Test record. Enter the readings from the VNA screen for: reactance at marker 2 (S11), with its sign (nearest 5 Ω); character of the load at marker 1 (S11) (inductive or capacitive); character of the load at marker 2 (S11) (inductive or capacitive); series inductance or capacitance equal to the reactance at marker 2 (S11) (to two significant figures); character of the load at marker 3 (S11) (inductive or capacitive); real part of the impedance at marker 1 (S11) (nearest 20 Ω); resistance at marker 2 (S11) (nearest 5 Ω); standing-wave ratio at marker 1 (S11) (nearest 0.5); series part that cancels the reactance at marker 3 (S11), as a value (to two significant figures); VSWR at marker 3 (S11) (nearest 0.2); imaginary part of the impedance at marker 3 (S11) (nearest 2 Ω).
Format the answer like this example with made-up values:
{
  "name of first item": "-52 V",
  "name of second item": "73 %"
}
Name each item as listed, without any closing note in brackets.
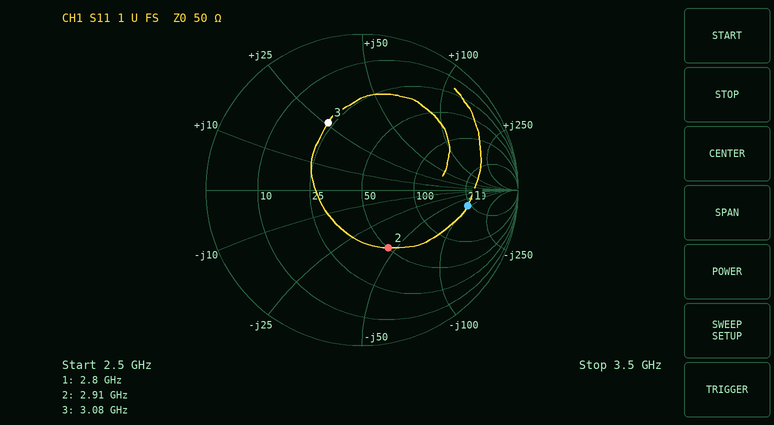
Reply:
{
  "reactance at marker 2 (S11), with its sign": "-45 Ω",
  "character of the load at marker 1 (S11)": "capacitive",
  "character of the load at marker 2 (S11)": "capacitive",
  "series inductance or capacitance equal to the reactance at marker 2 (S11)": "1.2 pF",
  "character of the load at marker 3 (S11)": "inductive",
  "real part of the impedance at marker 1 (S11)": "240 Ω",
  "resistance at marker 2 (S11)": "50 Ω",
  "standing-wave ratio at marker 1 (S11)": "5.5",
  "series part that cancels the reactance at marker 3 (S11), as a value": "2.0 pF",
  "VSWR at marker 3 (S11)": "2.8",
  "imaginary part of the impedance at marker 3 (S11)": "+26 Ω"
}
